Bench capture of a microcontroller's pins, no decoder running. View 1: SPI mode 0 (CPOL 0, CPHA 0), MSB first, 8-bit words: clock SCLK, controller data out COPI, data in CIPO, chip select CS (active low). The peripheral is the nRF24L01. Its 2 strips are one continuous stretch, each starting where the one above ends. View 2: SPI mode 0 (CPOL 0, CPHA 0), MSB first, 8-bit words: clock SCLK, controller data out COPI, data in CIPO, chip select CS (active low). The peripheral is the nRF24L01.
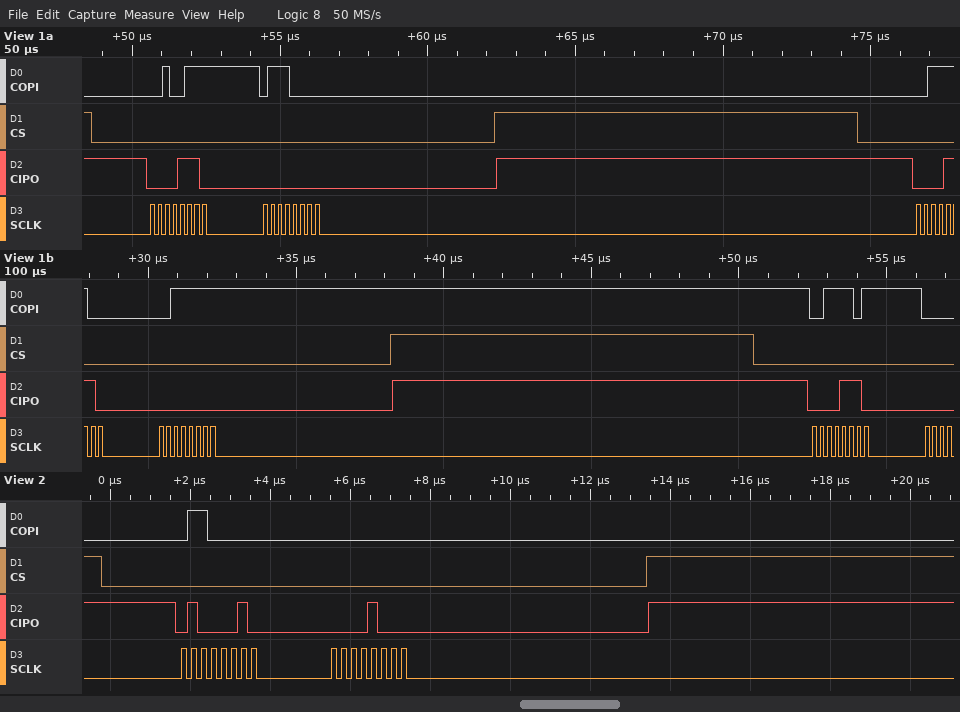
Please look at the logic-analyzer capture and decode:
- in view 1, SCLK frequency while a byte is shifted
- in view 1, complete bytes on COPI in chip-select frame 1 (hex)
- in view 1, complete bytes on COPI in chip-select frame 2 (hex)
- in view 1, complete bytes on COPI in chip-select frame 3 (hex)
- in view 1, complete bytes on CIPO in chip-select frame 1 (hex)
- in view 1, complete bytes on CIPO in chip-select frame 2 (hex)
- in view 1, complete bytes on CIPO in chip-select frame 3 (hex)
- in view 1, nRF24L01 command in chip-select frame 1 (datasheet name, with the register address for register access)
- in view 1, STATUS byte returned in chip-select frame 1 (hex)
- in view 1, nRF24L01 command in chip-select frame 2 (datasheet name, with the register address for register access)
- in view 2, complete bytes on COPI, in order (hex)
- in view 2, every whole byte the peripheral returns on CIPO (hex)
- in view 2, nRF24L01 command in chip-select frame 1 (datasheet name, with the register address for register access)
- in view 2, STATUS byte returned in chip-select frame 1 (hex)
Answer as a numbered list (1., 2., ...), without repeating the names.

1. 4 MHz
2. 0x27 0x70
3. 0x3C 0x3F
4. 0x3D
5. 0x0E 0x00
6. 0x0E 0x00
7. 0x0E
8. W_REGISTER 0x07
9. 0x0E
10. W_REGISTER 0x1C
11. 60 00
12. 42 08
13. R_RX_PL_WID
14. 0x42
